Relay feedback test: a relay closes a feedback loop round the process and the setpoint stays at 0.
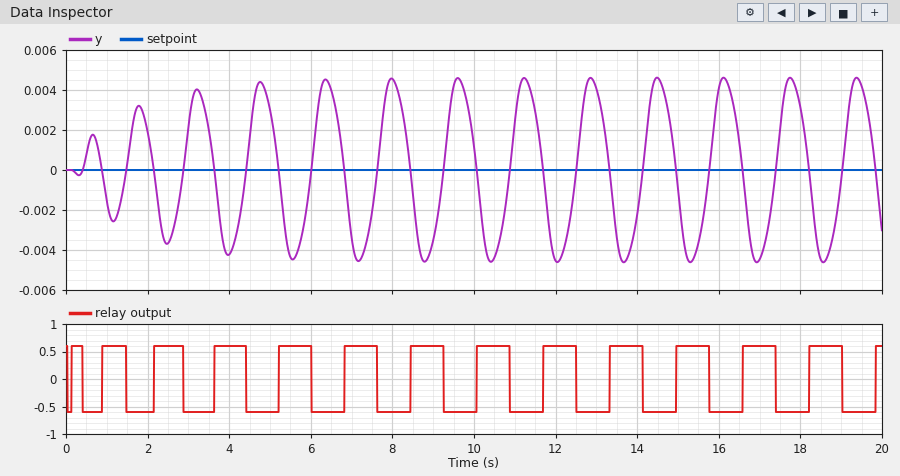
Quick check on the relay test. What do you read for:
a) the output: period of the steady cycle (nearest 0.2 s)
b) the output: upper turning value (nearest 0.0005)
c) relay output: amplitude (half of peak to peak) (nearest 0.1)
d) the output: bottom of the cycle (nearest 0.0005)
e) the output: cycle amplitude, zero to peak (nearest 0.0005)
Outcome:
1.6 s
0.0045
0.6
-0.0045
0.0045
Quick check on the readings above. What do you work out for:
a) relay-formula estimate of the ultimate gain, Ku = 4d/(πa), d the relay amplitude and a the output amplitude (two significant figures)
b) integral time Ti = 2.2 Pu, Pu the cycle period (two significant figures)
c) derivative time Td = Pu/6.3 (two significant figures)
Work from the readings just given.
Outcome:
170
3.5 s
0.25 s
